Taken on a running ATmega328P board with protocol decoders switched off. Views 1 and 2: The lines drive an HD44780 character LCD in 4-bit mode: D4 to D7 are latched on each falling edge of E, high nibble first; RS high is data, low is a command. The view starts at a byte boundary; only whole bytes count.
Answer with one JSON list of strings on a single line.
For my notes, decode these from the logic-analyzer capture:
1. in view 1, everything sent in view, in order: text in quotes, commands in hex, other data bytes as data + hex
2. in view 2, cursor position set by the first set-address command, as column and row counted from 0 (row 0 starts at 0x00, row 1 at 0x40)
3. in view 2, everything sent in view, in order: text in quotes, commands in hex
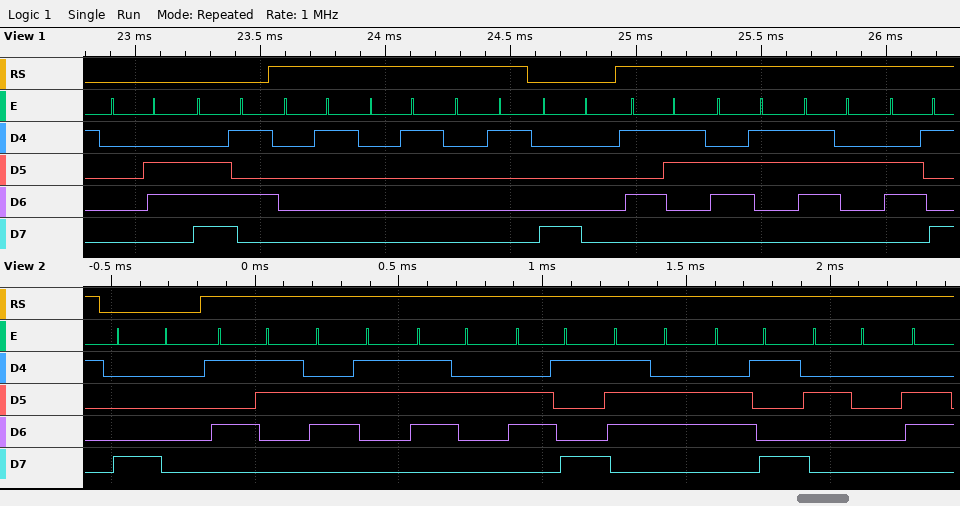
["0x06 0xE5 data 01 01 01 0x80 \"Scri\"", "column 0, row 0", "0x80 \"Scrivi \""]
